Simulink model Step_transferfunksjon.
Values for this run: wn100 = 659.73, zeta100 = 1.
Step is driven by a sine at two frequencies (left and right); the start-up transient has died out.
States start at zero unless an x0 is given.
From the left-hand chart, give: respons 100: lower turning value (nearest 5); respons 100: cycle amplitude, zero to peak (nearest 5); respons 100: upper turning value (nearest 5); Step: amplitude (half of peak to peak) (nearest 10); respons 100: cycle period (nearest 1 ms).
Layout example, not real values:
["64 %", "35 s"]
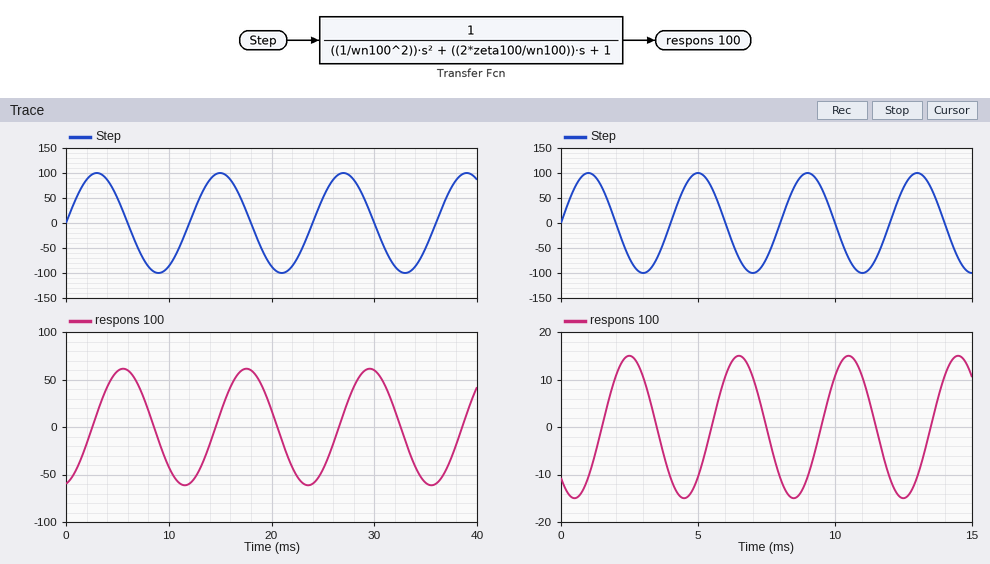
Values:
["-60", "60", "60", "100", "12 ms"]
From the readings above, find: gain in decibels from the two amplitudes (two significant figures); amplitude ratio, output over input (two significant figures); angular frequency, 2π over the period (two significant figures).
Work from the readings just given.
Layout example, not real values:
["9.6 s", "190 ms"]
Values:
["-4.4 dB", "0.60", "0.52 rad/ms"]
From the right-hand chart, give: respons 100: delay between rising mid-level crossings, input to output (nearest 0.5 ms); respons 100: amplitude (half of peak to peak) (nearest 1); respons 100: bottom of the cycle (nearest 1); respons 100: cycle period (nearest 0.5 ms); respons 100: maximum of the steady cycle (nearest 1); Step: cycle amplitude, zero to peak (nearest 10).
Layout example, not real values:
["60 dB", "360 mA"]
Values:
["1.5 ms", "15", "-15", "4.0 ms", "15", "100"]
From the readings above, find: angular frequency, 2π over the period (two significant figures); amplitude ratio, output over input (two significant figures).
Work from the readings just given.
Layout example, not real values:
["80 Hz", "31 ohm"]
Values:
["1.6 rad/ms", "0.15"]
